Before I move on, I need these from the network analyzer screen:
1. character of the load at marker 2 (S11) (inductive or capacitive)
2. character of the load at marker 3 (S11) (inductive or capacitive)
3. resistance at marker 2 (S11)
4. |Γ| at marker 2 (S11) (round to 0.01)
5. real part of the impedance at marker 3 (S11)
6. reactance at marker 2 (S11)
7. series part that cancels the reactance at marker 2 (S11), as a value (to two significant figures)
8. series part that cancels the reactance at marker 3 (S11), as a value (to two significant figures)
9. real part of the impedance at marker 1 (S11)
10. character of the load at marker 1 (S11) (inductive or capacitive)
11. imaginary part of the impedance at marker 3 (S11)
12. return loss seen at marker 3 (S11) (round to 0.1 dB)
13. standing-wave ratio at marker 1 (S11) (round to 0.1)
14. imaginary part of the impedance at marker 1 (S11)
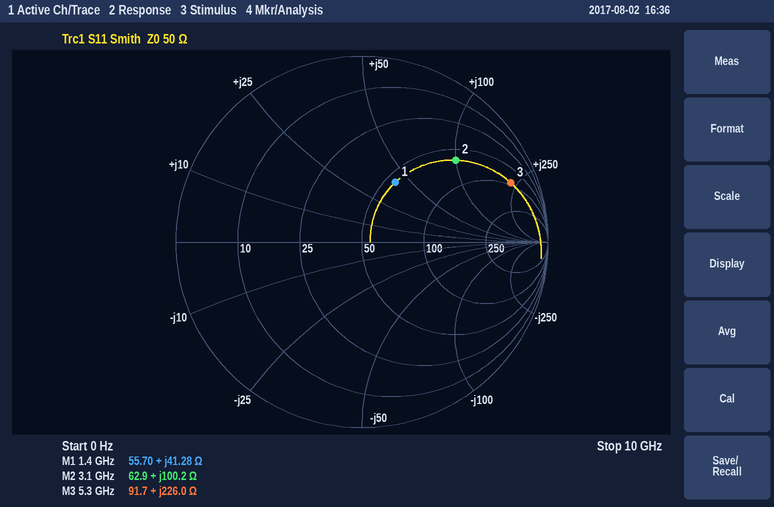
inductive
inductive
62.9 Ω
0.67
91.7 Ω
+100.2 Ω
510 fF
130 fF
55.70 Ω
inductive
+226.0 Ω
1.3 dB
2.2
+41.28 Ω
